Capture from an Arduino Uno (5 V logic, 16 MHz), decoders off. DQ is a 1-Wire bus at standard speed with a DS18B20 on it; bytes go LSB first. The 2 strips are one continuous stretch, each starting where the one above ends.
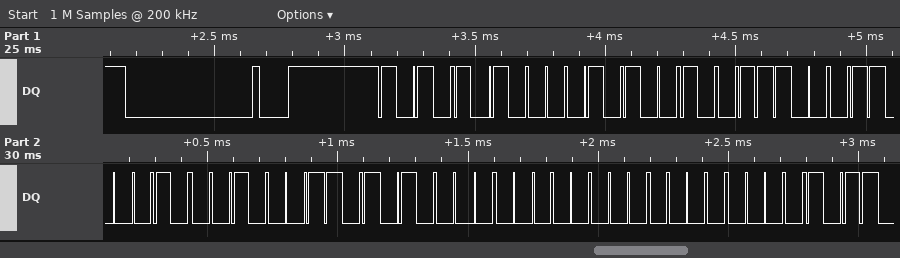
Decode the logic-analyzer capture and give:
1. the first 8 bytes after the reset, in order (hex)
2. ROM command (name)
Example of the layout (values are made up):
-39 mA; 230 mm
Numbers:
55 28 39 46 C4 0A 00 00; Match ROM
